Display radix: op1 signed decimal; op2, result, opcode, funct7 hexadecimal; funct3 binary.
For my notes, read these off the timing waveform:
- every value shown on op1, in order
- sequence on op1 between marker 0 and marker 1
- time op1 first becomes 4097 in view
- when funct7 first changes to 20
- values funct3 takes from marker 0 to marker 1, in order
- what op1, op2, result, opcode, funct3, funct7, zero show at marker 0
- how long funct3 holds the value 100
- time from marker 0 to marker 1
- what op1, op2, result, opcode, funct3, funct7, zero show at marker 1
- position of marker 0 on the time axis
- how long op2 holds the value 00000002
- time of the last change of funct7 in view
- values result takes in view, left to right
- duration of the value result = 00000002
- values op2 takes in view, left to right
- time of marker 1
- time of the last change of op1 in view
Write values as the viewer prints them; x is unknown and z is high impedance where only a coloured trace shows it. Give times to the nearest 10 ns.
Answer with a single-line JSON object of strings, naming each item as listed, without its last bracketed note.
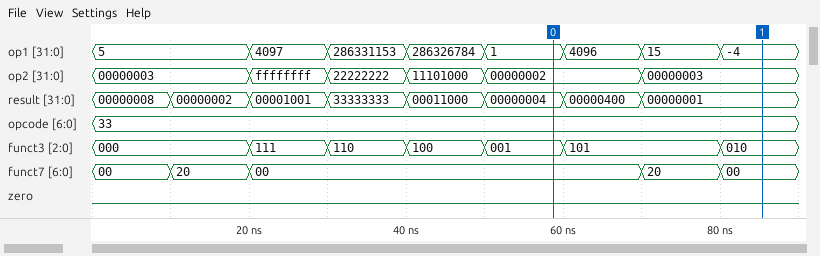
{"every value shown on op1, in order": "5, 4097, 286331153, 286326784, 1, 4096, 15, -4", "sequence on op1 between marker 0 and marker 1": "1, 4096, 15, -4", "time op1 first becomes 4097 in view": "20 ns", "when funct7 first changes to 20": "10 ns", "values funct3 takes from marker 0 to marker 1, in order": "001, 101, 010", "what op1, op2, result, opcode, funct3, funct7, zero show at marker 0": "op1=1, op2=00000002, result=00000004, opcode=33, funct3=001, funct7=00, zero=0", "how long funct3 holds the value 100": "10 ns", "time from marker 0 to marker 1": "30 ns", "what op1, op2, result, opcode, funct3, funct7, zero show at marker 1": "op1=-4, op2=00000003, result=00000001, opcode=33, funct3=010, funct7=00, zero=0", "position of marker 0 on the time axis": "60 ns", "how long op2 holds the value 00000002": "20 ns", "time of the last change of funct7 in view": "80 ns", "values result takes in view, left to right": "00000008, 00000002, 00001001, 33333333, 00011000, 00000004, 00000400, 00000001", "duration of the value result = 00000002": "10 ns", "values op2 takes in view, left to right": "00000003, ffffffff, 22222222, 11101000, 00000002, 00000003", "time of marker 1": "90 ns", "time of the last change of op1 in view": "80 ns"}
